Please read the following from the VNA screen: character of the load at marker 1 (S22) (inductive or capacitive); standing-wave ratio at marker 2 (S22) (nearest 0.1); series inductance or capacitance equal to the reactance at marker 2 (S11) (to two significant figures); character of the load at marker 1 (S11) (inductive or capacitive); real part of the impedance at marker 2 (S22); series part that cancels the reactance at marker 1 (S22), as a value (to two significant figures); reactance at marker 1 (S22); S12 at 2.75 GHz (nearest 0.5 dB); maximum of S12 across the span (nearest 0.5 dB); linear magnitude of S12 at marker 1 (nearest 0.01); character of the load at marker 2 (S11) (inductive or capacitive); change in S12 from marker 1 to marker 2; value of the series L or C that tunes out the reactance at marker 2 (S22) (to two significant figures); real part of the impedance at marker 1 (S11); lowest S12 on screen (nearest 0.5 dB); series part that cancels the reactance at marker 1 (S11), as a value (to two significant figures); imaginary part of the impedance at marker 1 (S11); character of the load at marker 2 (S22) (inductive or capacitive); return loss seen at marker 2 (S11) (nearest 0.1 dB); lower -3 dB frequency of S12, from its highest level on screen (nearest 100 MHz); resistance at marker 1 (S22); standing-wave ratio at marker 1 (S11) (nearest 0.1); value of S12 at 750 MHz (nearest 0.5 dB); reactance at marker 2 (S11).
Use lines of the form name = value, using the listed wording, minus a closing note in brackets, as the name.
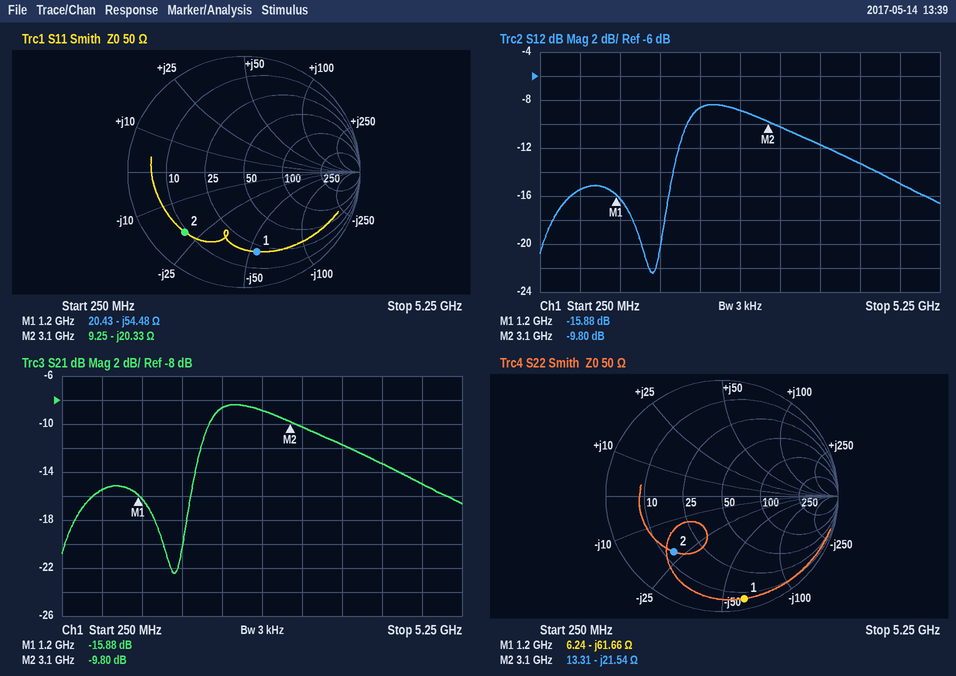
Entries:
character of the load at marker 1 (S22) = capacitive
standing-wave ratio at marker 2 (S22) = 4.5
series inductance or capacitance equal to the reactance at marker 2 (S11) = 2.5 pF
character of the load at marker 1 (S11) = capacitive
real part of the impedance at marker 2 = 13.31 Ω
series part that cancels the reactance at marker 1 (S22), as a value = 8.2 nH
reactance at marker 1 = -61.66 Ω
S12 at 2.75 GHz = -9.0 dB
maximum of S12 across the span = -8.5 dB
linear magnitude of S12 at marker 1 = 0.16
character of the load at marker 2 (S11) = capacitive
change in S12 from marker 1 to marker 2 = 6.08 dB
value of the series L or C that tunes out the reactance at marker 2 (S22) = 1.1 nH
real part of the impedance at marker 1 = 20.43 Ω
lowest S12 on screen = -22.5 dB
series part that cancels the reactance at marker 1 (S11), as a value = 7.2 nH
imaginary part of the impedance at marker 1 = -54.48 Ω
character of the load at marker 2 (S22) = capacitive
return loss seen at marker 2 (S11) = 2.8 dB
lower -3 dB frequency of S12, from its highest level on screen = 2.0 GHz
resistance at marker 1 = 6.24 Ω
standing-wave ratio at marker 1 (S11) = 5.6
value of S12 at 750 MHz = -15.5 dB
reactance at marker 2 = -20.33 Ω
